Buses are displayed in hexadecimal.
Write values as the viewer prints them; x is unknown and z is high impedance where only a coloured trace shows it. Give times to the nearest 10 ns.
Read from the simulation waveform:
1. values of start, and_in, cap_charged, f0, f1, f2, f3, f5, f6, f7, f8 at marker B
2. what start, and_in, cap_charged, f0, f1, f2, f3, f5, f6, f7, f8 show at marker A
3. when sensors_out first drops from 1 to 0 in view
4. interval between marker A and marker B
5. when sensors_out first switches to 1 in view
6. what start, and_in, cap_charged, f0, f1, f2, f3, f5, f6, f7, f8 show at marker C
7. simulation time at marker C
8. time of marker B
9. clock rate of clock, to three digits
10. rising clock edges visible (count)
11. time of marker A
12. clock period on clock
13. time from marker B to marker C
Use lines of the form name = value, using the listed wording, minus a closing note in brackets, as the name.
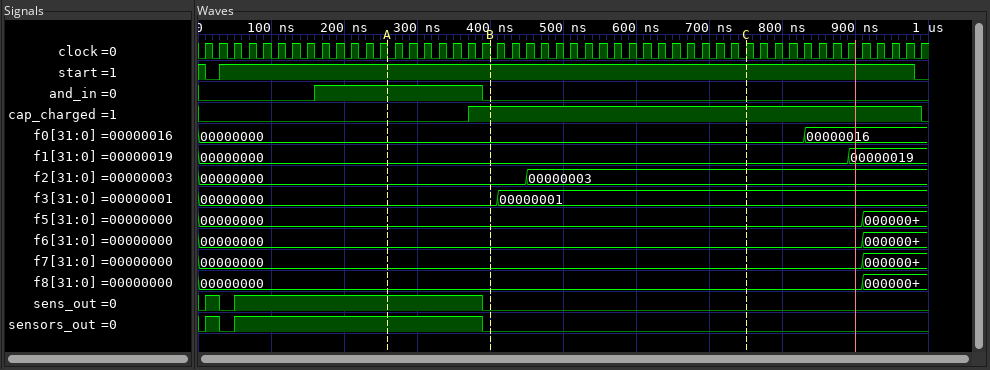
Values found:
values of start, and_in, cap_charged, f0, f1, f2, f3, f5, f6, f7, f8 at marker B = start=1, and_in=0, cap_charged=1, f0=00000000, f1=00000000, f2=00000000, f3=00000000, f5=00000000, f6=00000000, f7=00000000, f8=00000000
what start, and_in, cap_charged, f0, f1, f2, f3, f5, f6, f7, f8 show at marker A = start=1, and_in=1, cap_charged=0, f0=00000000, f1=00000000, f2=00000000, f3=00000000, f5=00000000, f6=00000000, f7=00000000, f8=00000000
when sensors_out first drops from 1 to 0 in view = 30 ns
interval between marker A and marker B = 140 ns
when sensors_out first switches to 1 in view = 10 ns
what start, and_in, cap_charged, f0, f1, f2, f3, f5, f6, f7, f8 show at marker C = start=1, and_in=0, cap_charged=1, f0=00000000, f1=00000000, f2=00000003, f3=00000001, f5=00000000, f6=00000000, f7=00000000, f8=00000000
simulation time at marker C = 750 ns
time of marker B = 400 ns
clock rate of clock, to three digits = 50.0 MHz
rising clock edges visible = 50
time of marker A = 260 ns
clock period on clock = 20 ns
time from marker B to marker C = 350 ns
